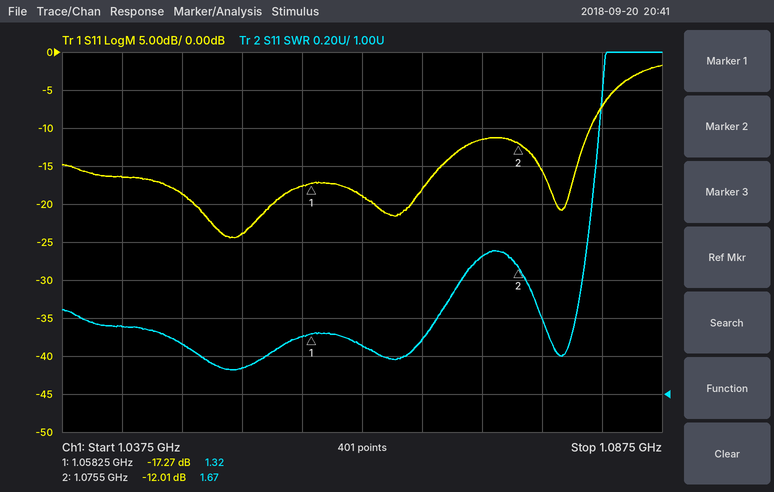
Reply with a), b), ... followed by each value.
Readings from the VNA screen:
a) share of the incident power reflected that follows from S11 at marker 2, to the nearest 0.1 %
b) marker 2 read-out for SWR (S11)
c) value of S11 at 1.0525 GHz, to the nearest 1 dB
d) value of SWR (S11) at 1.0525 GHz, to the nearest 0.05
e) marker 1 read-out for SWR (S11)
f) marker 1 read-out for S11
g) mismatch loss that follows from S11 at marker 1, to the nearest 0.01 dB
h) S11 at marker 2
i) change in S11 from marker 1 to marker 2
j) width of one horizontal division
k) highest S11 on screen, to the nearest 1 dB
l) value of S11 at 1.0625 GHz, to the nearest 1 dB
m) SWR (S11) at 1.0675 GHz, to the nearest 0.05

a) 6.3 %
b) 1.67
c) -24 dB
d) 1.15
e) 1.32
f) -17.27 dB
g) 0.08 dB
h) -12.01 dB
i) 5.26 dB
j) 5 MHz
k) -2 dB
l) -19 dB
m) 1.30
